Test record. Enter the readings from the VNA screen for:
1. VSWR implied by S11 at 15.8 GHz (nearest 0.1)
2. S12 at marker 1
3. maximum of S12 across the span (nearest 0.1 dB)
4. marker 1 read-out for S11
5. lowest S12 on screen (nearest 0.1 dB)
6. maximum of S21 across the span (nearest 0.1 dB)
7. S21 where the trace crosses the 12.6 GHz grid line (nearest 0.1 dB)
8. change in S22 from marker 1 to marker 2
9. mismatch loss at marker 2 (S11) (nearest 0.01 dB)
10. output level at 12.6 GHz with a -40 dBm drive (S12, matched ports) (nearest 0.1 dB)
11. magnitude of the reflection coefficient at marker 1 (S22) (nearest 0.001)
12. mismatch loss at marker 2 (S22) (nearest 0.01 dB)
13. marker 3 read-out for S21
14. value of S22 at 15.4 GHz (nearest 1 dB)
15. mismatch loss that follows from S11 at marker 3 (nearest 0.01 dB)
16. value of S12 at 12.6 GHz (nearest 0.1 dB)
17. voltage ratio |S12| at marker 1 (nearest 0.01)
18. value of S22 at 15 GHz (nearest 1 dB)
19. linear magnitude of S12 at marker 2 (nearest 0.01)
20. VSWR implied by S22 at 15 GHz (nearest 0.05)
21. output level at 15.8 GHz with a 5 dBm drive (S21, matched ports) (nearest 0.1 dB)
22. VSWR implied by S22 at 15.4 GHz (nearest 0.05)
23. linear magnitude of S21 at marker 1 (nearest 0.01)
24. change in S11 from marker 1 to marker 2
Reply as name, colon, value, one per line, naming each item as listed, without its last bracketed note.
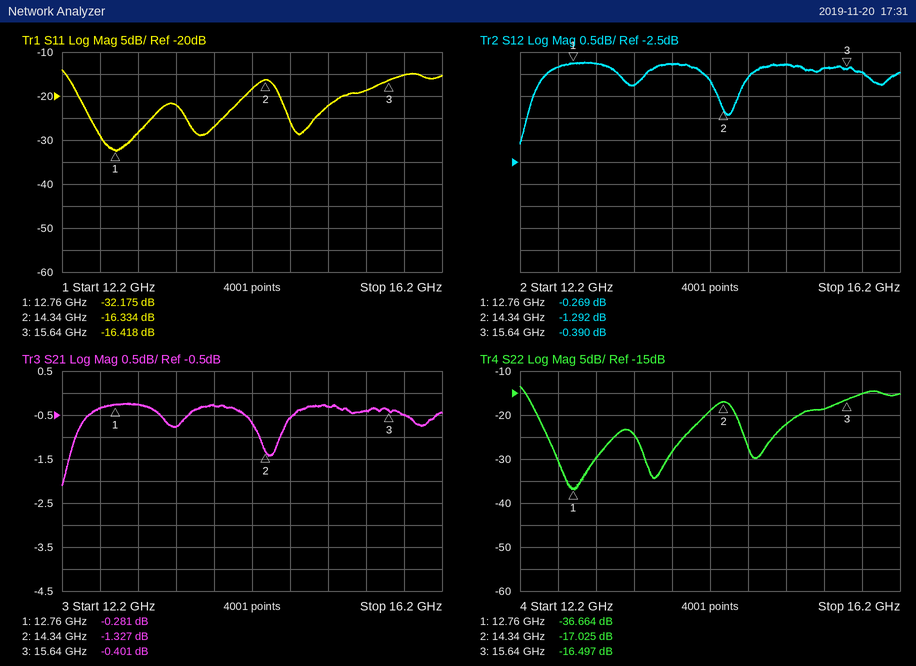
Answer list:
VSWR implied by S11 at 15.8 GHz: 1.4
S12 at marker 1: -0.269 dB
maximum of S12 across the span: -0.2 dB
marker 1 read-out for S11: -32.175 dB
lowest S12 on screen: -2.1 dB
maximum of S21 across the span: -0.2 dB
S21 where the trace crosses the 12.6 GHz grid line: -0.3 dB
change in S22 from marker 1 to marker 2: 19.639 dB
mismatch loss at marker 2 (S11): 0.10 dB
output level at 12.6 GHz with a -40 dBm drive (S12, matched ports): -40.3 dBm
magnitude of the reflection coefficient at marker 1 (S22): 0.015
mismatch loss at marker 2 (S22): 0.09 dB
marker 3 read-out for S21: -0.401 dB
value of S22 at 15.4 GHz: -19 dB
mismatch loss that follows from S11 at marker 3: 0.10 dB
value of S12 at 12.6 GHz: -0.3 dB
voltage ratio |S12| at marker 1: 0.97
value of S22 at 15 GHz: -22 dB
linear magnitude of S12 at marker 2: 0.86
VSWR implied by S22 at 15 GHz: 1.15
output level at 15.8 GHz with a 5 dBm drive (S21, matched ports): 4.5 dBm
VSWR implied by S22 at 15.4 GHz: 1.25
linear magnitude of S21 at marker 1: 0.97
change in S11 from marker 1 to marker 2: 15.841 dB
